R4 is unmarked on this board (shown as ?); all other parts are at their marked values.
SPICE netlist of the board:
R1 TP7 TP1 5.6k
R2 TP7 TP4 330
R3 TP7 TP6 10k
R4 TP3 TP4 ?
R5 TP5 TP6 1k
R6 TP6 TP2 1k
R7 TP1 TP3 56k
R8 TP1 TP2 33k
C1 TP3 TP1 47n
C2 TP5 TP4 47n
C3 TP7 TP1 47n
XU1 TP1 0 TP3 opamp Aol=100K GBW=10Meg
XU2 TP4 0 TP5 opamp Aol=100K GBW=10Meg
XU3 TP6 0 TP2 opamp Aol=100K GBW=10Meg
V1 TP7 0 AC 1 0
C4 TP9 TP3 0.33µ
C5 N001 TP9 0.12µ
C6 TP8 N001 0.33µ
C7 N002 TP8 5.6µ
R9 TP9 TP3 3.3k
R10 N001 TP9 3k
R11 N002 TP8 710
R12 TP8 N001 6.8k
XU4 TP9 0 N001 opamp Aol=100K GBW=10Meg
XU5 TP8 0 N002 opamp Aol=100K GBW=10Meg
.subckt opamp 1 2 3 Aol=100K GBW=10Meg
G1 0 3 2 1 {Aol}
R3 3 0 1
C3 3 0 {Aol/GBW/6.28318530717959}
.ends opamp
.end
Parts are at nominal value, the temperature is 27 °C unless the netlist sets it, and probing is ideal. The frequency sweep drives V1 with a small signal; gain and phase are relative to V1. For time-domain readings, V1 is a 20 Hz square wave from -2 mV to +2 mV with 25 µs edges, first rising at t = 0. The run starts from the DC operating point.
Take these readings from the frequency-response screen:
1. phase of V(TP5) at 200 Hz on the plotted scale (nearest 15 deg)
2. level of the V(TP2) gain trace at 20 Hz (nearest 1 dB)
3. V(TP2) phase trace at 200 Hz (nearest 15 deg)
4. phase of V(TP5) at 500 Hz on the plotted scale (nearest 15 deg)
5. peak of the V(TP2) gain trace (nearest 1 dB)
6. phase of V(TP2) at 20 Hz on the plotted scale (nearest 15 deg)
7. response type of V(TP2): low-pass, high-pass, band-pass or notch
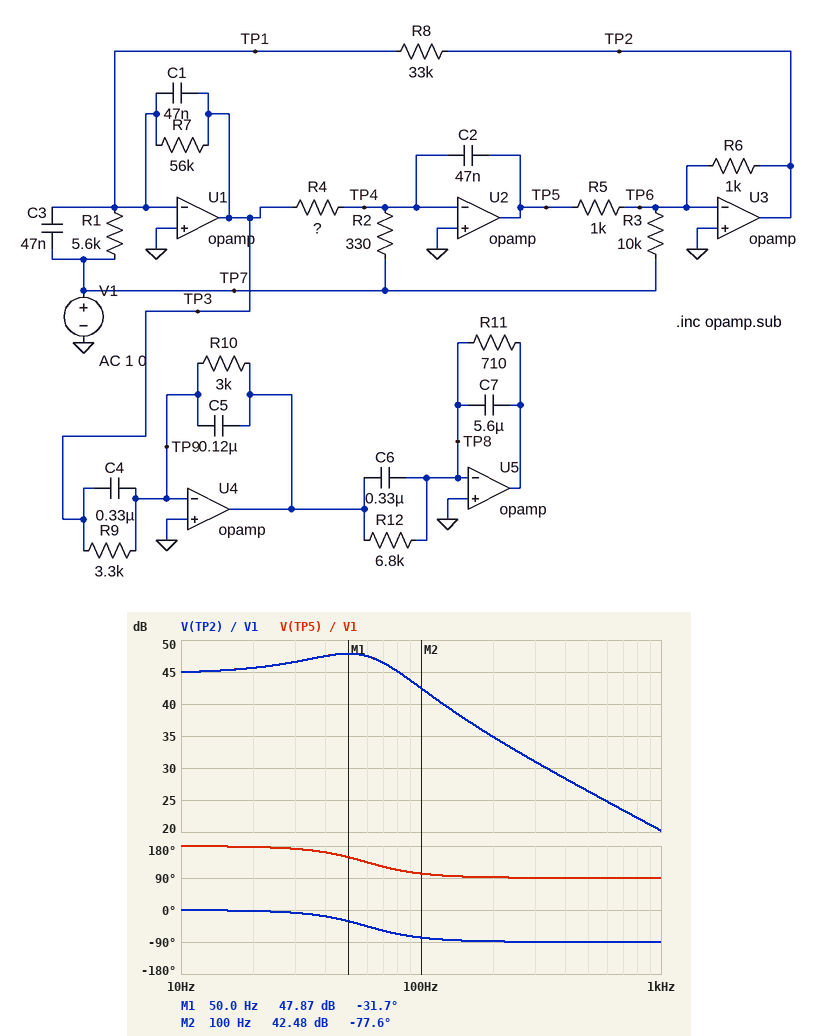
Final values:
90 deg
46 dB
-90 deg
90 deg
48 dB
0 deg
low-pass
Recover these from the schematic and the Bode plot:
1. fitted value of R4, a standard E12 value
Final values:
100 kΩ
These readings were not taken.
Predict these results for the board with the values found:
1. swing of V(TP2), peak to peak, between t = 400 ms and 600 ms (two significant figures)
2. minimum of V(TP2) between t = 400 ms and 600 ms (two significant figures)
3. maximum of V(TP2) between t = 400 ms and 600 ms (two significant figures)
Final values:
1.1 V
-540 mV
540 mV
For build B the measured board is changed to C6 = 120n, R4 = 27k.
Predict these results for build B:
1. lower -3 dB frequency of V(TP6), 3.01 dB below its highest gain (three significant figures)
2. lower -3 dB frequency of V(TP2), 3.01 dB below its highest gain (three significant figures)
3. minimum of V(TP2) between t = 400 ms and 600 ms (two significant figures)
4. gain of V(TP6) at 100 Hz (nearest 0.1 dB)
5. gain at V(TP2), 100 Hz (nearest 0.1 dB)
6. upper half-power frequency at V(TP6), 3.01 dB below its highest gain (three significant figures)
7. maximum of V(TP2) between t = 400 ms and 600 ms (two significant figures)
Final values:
90.3 Hz
84.1 Hz
-300 mV
-52.3 dB
44.7 dB
162 Hz
300 mV
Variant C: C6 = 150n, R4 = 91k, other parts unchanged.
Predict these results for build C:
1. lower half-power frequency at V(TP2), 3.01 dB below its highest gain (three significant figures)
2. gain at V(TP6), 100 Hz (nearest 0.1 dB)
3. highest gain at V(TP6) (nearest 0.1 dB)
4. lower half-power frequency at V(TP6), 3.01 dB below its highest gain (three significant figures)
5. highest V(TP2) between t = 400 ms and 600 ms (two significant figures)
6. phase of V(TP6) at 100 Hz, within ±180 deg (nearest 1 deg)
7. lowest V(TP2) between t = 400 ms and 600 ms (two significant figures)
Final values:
17.2 Hz
-54.3 dB
-51.2 dB
26.7 Hz
520 mV
149 deg
-520 mV
